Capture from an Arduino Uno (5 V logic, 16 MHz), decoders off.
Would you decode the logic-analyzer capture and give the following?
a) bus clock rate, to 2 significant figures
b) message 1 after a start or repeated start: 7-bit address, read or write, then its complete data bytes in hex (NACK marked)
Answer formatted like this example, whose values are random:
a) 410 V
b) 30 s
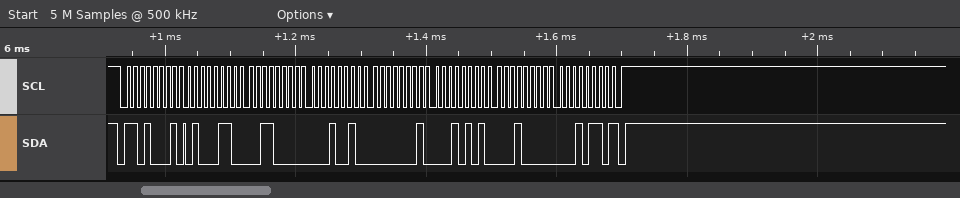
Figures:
a) 100 kHz
b) 0x68 read: 46 30 12 01 15 10 16 NACK
